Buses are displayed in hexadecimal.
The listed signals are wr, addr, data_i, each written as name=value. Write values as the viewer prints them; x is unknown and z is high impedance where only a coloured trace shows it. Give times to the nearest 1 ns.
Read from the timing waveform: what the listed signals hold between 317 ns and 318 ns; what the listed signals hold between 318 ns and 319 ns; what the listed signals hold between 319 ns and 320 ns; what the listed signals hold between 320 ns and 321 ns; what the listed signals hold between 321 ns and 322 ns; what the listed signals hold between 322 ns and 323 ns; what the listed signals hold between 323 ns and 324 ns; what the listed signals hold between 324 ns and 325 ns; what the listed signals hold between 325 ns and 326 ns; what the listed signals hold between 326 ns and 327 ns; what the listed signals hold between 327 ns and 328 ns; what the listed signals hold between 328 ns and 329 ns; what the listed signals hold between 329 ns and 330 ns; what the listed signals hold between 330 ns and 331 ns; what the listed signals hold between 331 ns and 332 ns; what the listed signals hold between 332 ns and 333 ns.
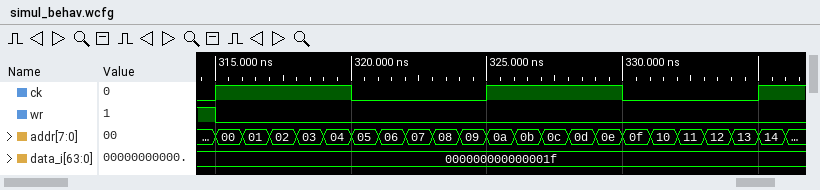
wr=0, addr=02, data_i=000000000000001f
wr=0, addr=03, data_i=000000000000001f
wr=0, addr=04, data_i=000000000000001f
wr=0, addr=05, data_i=000000000000001f
wr=0, addr=06, data_i=000000000000001f
wr=0, addr=07, data_i=000000000000001f
wr=0, addr=08, data_i=000000000000001f
wr=0, addr=09, data_i=000000000000001f
wr=0, addr=0a, data_i=000000000000001f
wr=0, addr=0b, data_i=000000000000001f
wr=0, addr=0c, data_i=000000000000001f
wr=0, addr=0d, data_i=000000000000001f
wr=0, addr=0e, data_i=000000000000001f
wr=0, addr=0f, data_i=000000000000001f
wr=0, addr=10, data_i=000000000000001f
wr=0, addr=11, data_i=000000000000001f
